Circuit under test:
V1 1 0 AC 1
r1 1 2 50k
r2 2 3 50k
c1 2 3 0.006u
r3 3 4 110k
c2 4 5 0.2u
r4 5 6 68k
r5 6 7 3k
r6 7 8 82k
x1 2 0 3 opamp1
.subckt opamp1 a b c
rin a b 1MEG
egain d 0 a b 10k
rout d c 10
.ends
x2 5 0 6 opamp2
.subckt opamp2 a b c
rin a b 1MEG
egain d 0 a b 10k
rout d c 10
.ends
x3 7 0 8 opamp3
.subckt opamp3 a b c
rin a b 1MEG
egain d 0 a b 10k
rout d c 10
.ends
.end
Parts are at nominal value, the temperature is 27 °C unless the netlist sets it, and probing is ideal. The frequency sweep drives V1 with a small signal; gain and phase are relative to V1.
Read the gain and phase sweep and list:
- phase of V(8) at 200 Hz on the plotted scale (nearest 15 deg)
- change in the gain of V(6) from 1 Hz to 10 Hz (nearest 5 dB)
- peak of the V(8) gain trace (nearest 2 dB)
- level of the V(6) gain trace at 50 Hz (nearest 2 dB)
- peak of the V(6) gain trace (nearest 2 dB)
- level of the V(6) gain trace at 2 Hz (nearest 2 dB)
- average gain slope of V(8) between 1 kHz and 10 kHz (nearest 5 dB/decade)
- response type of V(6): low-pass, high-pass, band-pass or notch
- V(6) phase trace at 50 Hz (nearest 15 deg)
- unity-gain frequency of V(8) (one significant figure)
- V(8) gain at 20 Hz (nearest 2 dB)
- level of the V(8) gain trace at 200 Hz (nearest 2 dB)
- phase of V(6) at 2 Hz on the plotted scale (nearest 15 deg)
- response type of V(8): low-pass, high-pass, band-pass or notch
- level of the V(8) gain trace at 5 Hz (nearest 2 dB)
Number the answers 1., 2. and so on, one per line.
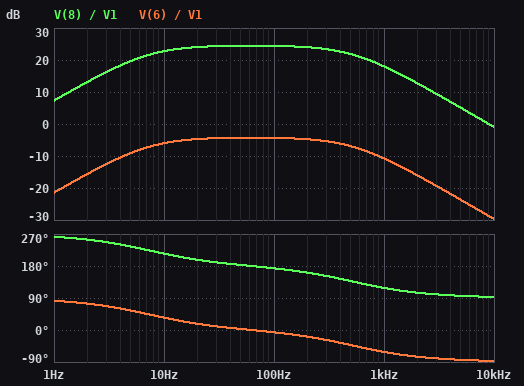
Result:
1. 165 deg
2. 15 dB
3. 24 dB
4. -4 dB
5. -4 dB
6. -16 dB
7. -20 dB/decade
8. band-pass
9. 0 deg
10. 9 kHz
11. 24 dB
12. 24 dB
13. 75 deg
14. band-pass
15. 20 dB
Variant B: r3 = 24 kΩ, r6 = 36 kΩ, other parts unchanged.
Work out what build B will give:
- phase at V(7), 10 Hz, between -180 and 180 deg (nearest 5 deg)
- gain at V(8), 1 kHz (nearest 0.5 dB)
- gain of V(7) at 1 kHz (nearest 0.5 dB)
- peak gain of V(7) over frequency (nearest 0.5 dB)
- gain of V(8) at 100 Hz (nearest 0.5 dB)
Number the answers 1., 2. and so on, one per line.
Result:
1. -110 deg
2. 24.0 dB
3. -56.0 dB
4. -50.0 dB
5. 30.0 dB
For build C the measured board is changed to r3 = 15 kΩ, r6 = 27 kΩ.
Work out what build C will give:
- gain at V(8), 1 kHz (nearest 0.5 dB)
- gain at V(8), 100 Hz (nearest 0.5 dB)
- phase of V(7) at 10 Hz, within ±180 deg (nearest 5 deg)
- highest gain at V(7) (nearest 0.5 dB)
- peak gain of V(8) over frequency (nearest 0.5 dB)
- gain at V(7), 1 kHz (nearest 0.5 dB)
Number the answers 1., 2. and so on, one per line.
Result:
1. 25.5 dB
2. 31.0 dB
3. -100 deg
4. -48.5 dB
5. 31.5 dB
6. -54.5 dB
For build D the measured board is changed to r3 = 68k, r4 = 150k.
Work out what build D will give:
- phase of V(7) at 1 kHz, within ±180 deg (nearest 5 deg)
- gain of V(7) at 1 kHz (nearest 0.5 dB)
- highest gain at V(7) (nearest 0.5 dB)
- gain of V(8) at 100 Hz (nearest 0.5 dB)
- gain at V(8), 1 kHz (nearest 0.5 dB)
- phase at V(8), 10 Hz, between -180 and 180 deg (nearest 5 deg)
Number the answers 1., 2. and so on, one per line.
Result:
1. 120 deg
2. -51.0 dB
3. -44.5 dB
4. 35.5 dB
5. 29.0 dB
6. -130 deg
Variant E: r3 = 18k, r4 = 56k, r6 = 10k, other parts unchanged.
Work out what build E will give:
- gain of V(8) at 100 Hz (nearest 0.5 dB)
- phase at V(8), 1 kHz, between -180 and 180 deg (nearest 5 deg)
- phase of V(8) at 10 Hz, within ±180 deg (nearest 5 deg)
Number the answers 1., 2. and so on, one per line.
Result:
1. 19.5 dB
2. 120 deg
3. -105 deg
